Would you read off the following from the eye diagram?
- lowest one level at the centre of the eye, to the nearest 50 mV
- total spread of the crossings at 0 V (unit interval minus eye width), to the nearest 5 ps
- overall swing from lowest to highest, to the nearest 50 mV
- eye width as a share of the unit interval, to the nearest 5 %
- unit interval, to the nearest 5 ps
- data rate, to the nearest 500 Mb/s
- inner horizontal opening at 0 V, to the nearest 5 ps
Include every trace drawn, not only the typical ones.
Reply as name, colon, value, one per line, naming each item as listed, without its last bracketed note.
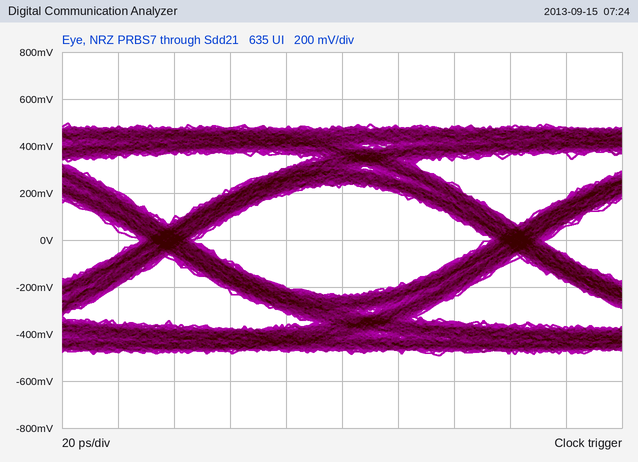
lowest one level at the centre of the eye, to the nearest 50 mV: 250 mV
total spread of the crossings at 0 V (unit interval minus eye width), to the nearest 5 ps: 20 ps
overall swing from lowest to highest, to the nearest 50 mV: 1.00 V
eye width as a share of the unit interval, to the nearest 5 %: 85 %
unit interval, to the nearest 5 ps: 125 ps
data rate, to the nearest 500 Mb/s: 8.0 Gb/s
inner horizontal opening at 0 V, to the nearest 5 ps: 105 ps
